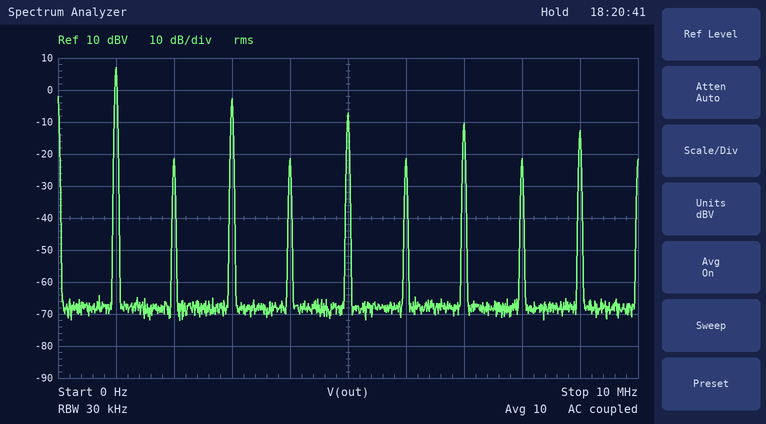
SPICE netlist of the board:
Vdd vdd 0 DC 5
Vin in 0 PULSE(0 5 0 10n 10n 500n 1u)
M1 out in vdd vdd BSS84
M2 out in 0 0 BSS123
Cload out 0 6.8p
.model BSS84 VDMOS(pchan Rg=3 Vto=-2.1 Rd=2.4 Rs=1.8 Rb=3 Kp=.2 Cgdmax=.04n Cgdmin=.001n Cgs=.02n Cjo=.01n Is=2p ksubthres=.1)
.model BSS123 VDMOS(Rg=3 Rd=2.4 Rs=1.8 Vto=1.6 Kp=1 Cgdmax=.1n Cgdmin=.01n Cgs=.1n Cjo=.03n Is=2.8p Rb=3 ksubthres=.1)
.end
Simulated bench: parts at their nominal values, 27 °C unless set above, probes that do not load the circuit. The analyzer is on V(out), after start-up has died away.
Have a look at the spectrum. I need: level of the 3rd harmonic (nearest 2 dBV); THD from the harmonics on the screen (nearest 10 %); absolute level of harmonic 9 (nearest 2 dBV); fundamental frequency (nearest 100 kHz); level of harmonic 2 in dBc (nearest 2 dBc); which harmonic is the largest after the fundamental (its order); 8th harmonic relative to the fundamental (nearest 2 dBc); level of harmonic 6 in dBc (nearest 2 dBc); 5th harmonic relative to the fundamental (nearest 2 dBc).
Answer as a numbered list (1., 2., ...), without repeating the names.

1. -2 dBV
2. 40 %
3. -12 dBV
4. 1.0 MHz
5. -28 dBc
6. 3
7. -28 dBc
8. -28 dBc
9. -14 dBc
